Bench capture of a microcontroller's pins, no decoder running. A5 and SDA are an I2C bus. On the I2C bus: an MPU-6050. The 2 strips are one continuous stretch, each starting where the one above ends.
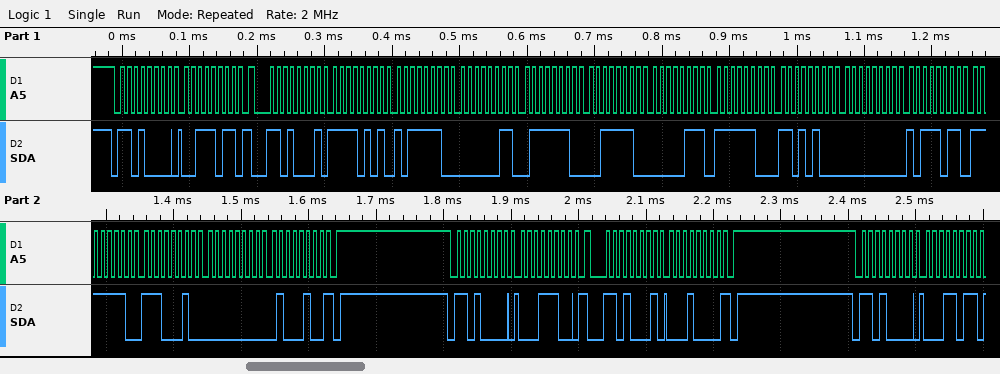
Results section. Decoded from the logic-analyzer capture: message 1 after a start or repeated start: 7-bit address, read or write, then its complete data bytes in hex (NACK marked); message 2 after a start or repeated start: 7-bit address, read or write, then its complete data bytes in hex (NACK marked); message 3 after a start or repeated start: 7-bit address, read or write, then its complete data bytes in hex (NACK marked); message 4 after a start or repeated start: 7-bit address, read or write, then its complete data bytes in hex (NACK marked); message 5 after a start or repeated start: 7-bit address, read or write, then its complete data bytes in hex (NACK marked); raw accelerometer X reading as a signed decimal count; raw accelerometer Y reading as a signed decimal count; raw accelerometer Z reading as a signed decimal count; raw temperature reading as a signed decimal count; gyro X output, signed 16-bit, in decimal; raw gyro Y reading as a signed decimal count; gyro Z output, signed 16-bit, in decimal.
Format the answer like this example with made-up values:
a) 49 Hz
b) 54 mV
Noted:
a) 0x68 write: 3B
b) 0x68 read: F5 BE 03 7E 3E 07 FC D4 00 BB FE E2 00 44 NACK
c) 0x68 write: 1C
d) 0x68 read: 10 NACK
e) 0x68 write: 1B
f) -2626
g) 894
h) 15879
i) -812
j) 187
k) -286
l) 68
